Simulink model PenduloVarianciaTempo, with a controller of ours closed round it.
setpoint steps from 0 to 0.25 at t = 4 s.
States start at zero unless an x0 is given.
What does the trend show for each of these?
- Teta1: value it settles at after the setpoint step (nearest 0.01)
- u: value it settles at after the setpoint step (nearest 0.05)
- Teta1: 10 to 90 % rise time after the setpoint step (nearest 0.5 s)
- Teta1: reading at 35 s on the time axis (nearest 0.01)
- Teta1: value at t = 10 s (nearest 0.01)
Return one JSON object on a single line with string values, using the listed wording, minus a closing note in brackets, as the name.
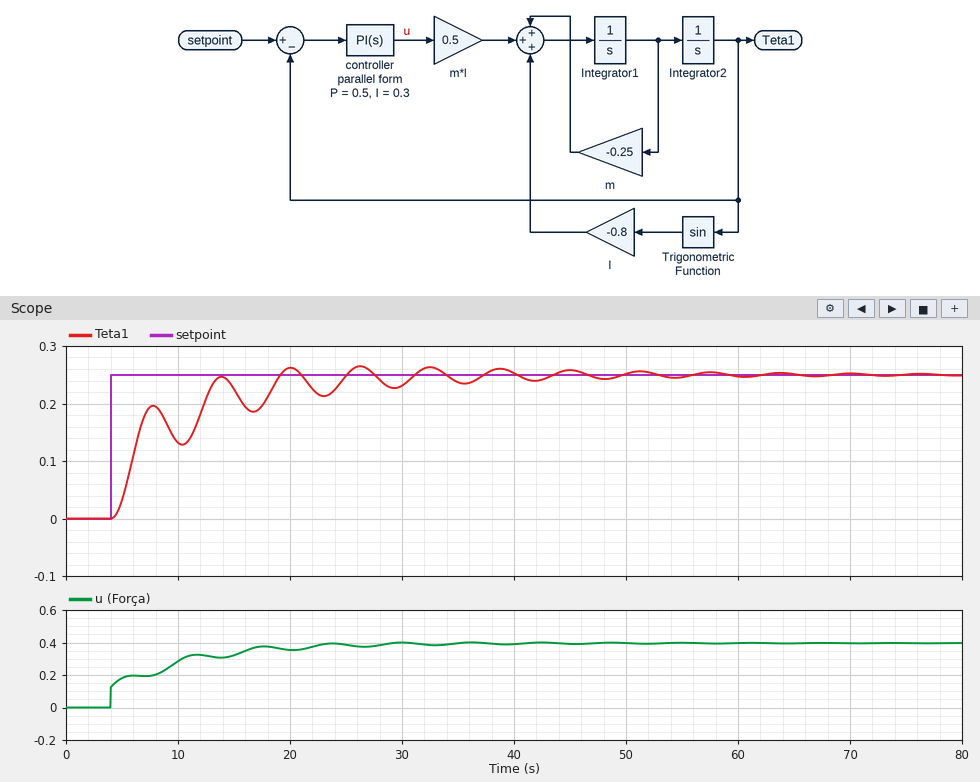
{"Teta1: value it settles at after the setpoint step": "0.25", "u: value it settles at after the setpoint step": "0.40", "Teta1: 10 to 90 % rise time after the setpoint step": "8.0 s", "Teta1: reading at 35 s on the time axis": "0.24", "Teta1: value at t = 10 s": "0.13"}
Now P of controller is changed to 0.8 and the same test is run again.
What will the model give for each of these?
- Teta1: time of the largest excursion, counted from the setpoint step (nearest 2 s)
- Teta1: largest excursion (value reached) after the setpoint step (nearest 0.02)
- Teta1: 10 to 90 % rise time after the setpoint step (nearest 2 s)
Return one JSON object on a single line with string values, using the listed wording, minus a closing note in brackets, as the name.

{"Teta1: time of the largest excursion, counted from the setpoint step": "20 s", "Teta1: largest excursion (value reached) after the setpoint step": "0.26", "Teta1: 10 to 90 % rise time after the setpoint step": "8 s"}
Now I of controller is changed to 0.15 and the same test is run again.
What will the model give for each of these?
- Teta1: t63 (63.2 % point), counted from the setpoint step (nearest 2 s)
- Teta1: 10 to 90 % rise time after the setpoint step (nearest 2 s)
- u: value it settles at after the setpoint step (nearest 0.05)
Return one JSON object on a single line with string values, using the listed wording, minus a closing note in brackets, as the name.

{"Teta1: t63 (63.2 % point), counted from the setpoint step": "8 s", "Teta1: 10 to 90 % rise time after the setpoint step": "26 s", "u: value it settles at after the setpoint step": "0.40"}
